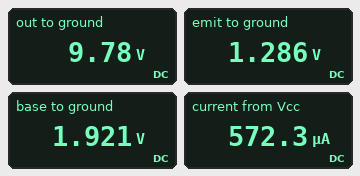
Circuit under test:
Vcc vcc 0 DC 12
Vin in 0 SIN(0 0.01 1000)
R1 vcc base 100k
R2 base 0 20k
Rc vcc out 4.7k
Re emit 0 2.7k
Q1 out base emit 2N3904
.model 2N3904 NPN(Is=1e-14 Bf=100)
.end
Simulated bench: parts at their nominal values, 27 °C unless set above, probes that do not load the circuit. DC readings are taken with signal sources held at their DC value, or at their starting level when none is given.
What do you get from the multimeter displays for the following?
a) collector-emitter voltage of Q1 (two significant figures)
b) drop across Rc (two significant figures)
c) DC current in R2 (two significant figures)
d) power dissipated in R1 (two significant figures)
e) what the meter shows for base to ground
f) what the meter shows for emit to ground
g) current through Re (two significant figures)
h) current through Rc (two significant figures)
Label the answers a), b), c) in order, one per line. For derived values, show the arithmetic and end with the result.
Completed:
a) 9.78 V - 1.286 V = 8.5 V
b) 12 V - 9.78 V = 2.2 V
c) (1.921 V) / 20 kΩ = 96 µA
d) (12 V - 1.921 V)^2 / 100 kΩ = 1.0 mW
e) 1.921 V
f) 1.286 V
g) (1.286 V) / 2.7 kΩ = 480 µA
h) (12 V - 9.78 V) / 4.7 kΩ = 470 µA
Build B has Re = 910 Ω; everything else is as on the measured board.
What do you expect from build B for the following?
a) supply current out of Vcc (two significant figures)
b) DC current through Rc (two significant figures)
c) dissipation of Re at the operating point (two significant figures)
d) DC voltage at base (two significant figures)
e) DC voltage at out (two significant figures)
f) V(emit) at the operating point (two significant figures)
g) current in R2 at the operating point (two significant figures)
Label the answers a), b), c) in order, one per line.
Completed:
a) 1.3 mA
b) 1.2 mA
c) 1.4 mW
d) 1.8 V
e) 6.2 V
f) 1.1 V
g) 90 µA
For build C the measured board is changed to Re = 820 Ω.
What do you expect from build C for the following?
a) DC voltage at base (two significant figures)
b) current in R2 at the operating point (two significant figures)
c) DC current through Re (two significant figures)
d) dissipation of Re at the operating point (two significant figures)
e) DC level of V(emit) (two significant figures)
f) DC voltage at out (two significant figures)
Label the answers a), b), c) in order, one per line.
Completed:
a) 1.8 V
b) 89 µA
c) 1.4 mA
d) 1.5 mW
e) 1.1 V
f) 5.7 V
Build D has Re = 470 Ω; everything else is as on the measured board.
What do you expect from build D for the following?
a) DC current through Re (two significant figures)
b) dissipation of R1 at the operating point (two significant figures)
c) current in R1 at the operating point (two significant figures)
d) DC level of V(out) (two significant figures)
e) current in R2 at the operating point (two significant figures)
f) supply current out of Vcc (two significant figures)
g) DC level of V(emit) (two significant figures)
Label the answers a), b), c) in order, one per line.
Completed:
a) 2.1 mA
b) 1.1 mW
c) 100 µA
d) 2.3 V
e) 83 µA
f) 2.2 mA
g) 980 mV
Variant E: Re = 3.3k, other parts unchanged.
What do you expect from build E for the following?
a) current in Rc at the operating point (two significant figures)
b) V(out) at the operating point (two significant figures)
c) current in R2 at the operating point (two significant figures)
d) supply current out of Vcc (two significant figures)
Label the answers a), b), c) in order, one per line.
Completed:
a) 390 µA
b) 10 V
c) 97 µA
d) 490 µA
